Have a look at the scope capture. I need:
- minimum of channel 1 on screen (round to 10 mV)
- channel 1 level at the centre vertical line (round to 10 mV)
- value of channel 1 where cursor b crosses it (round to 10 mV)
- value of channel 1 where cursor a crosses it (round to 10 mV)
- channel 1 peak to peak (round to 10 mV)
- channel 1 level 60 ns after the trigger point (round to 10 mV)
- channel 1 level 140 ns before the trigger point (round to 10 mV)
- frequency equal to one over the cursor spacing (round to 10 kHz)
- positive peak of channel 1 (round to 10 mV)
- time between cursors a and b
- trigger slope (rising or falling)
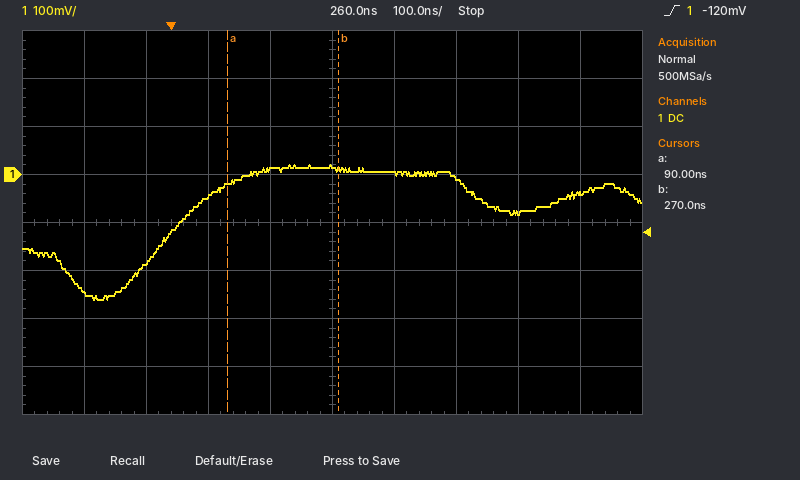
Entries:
-260 mV
20 mV
10 mV
-20 mV
280 mV
-50 mV
-240 mV
5.56 MHz
20 mV
180 ns
rising
